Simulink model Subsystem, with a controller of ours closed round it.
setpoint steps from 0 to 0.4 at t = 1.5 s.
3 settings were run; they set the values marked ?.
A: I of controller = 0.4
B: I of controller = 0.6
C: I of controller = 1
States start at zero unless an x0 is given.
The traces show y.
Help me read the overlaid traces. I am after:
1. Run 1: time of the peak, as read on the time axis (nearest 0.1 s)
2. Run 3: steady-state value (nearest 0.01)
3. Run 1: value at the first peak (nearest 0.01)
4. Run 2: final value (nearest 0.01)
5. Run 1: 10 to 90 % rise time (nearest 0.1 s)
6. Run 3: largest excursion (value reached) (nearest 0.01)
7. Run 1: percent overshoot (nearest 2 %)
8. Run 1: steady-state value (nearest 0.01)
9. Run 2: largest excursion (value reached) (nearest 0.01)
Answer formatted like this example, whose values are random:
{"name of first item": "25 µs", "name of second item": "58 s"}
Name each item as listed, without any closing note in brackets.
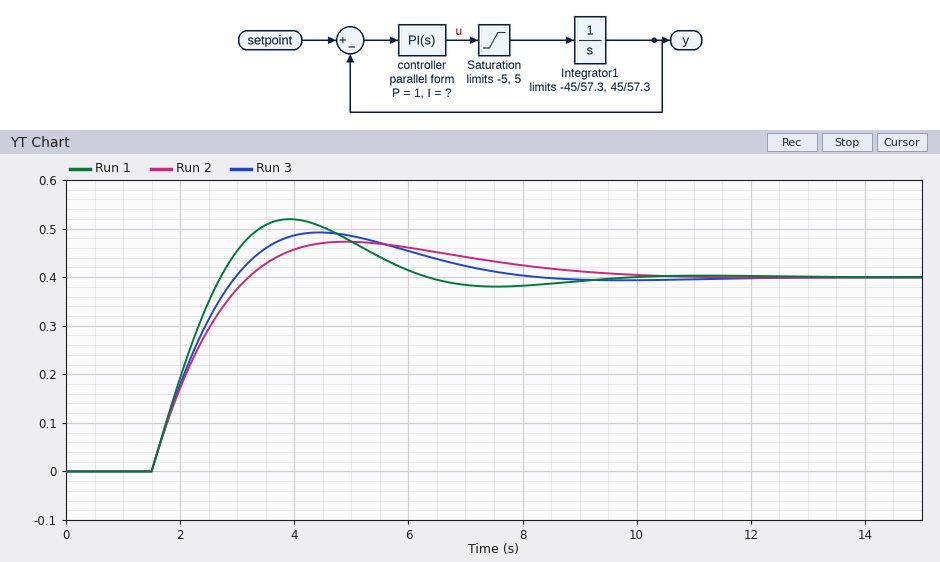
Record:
{"Run 1: time of the peak, as read on the time axis": "3.9 s", "Run 3: steady-state value": "0.40", "Run 1: value at the first peak": "0.52", "Run 2: final value": "0.40", "Run 1: 10 to 90 % rise time": "0.9 s", "Run 3: largest excursion (value reached)": "0.49", "Run 1: percent overshoot": "30 %", "Run 1: steady-state value": "0.40", "Run 2: largest excursion (value reached)": "0.47"}
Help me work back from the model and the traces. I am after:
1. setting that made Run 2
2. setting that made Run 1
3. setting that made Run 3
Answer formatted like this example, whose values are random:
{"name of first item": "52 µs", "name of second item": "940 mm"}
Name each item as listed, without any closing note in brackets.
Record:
{"setting that made Run 2": "A", "setting that made Run 1": "C", "setting that made Run 3": "B"}
